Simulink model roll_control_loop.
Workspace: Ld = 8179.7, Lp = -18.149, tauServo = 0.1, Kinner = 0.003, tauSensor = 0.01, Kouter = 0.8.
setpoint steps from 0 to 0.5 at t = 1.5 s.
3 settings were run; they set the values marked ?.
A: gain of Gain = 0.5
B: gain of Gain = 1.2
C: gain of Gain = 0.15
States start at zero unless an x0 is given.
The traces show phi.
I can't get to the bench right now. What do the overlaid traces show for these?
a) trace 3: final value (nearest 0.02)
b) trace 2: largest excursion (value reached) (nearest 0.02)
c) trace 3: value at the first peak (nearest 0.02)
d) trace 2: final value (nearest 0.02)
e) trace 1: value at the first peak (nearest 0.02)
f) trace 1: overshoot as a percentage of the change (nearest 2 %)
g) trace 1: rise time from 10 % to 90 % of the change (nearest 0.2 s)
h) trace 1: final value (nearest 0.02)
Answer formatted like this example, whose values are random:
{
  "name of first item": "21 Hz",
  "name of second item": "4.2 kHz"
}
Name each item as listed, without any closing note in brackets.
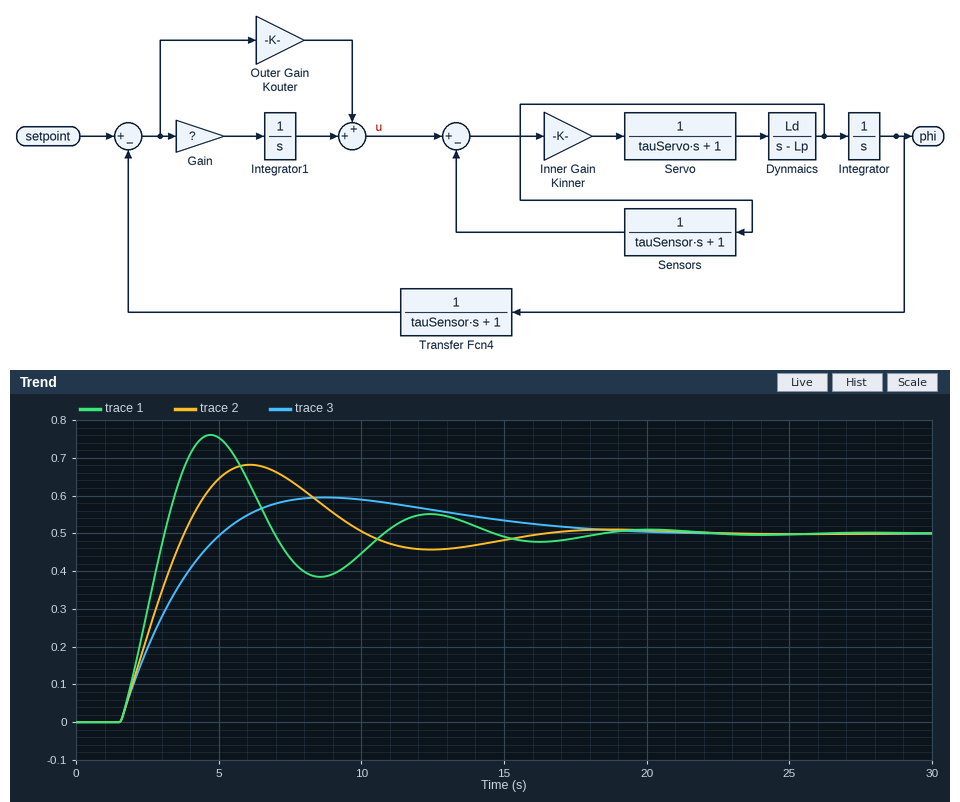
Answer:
{
  "trace 3: final value": "0.50",
  "trace 2: largest excursion (value reached)": "0.68",
  "trace 3: value at the first peak": "0.60",
  "trace 2: final value": "0.50",
  "trace 1: value at the first peak": "0.76",
  "trace 1: overshoot as a percentage of the change": "52 %",
  "trace 1: rise time from 10 % to 90 % of the change": "1.2 s",
  "trace 1: final value": "0.50"
}
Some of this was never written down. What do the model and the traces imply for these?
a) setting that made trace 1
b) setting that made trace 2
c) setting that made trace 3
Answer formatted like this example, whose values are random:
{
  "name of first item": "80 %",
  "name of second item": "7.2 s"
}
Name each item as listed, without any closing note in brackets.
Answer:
{
  "setting that made trace 1": "B",
  "setting that made trace 2": "A",
  "setting that made trace 3": "C"
}
